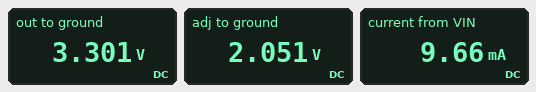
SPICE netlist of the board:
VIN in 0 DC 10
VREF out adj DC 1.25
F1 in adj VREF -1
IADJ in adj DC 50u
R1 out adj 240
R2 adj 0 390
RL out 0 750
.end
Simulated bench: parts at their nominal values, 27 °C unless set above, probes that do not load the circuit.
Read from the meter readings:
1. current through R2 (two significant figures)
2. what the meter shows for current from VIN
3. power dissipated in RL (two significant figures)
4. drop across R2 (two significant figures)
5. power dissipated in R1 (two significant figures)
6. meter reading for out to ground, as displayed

5.3 mA
9.66 mA
15 mW
2.1 V
6.5 mW
3.301 V
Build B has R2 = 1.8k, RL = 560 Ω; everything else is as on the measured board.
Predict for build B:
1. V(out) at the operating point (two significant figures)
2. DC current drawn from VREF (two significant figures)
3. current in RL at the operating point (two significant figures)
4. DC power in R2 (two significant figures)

11 V
24 mA
19 mA
50 mW
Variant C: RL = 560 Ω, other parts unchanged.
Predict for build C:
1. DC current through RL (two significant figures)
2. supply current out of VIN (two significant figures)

5.9 mA
11 mA
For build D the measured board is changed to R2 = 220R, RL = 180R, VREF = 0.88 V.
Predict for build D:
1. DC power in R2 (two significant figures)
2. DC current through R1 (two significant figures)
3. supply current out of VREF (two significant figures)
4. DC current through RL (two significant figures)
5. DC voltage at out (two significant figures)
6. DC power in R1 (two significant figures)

3.0 mW
3.7 mA
13 mA
9.4 mA
1.7 V
3.2 mW
